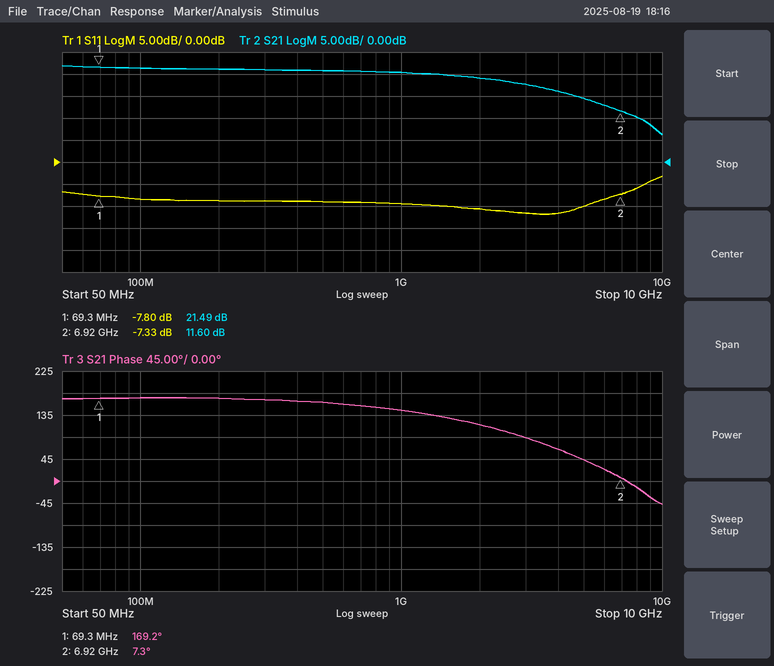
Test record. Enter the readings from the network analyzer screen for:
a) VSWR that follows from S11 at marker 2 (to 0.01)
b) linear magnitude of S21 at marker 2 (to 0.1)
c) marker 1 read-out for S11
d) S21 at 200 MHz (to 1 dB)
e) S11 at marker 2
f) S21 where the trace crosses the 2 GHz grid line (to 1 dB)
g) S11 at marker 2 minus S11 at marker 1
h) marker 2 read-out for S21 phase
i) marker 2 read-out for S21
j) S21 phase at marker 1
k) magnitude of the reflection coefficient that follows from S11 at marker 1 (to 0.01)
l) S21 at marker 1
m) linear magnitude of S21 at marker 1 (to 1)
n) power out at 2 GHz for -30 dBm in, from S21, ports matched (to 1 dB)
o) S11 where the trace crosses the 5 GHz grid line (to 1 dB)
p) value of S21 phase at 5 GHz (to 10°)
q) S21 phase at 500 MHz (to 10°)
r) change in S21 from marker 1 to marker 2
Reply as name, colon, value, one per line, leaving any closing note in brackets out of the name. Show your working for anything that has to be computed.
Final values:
VSWR that follows from S11 at marker 2: (1 + 0.4300)/(1 − 0.4300) ≈ 2.51
linear magnitude of S21 at marker 2: 10^(11.6/20) ≈ 3.8
marker 1 read-out for S11: -7.80 dB
S21 at 200 MHz: 21 dB
S11 at marker 2: -7.33 dB
S21 where the trace crosses the 2 GHz grid line: 19 dB
S11 at marker 2 minus S11 at marker 1: -7.33 − (-7.8) = 0.47 dB
marker 2 read-out for S21 phase: 7.3°
marker 2 read-out for S21: 11.60 dB
S21 phase at marker 1: 169.2°
magnitude of the reflection coefficient that follows from S11 at marker 1: 10^(-7.8/20) ≈ 0.41
S21 at marker 1: 21.49 dB
linear magnitude of S21 at marker 1: 10^(21.49/20) ≈ 12
power out at 2 GHz for -30 dBm in, from S21, ports matched: -30 dBm + (19 dB) = -11 dBm
S11 where the trace crosses the 5 GHz grid line: -10 dB
value of S21 phase at 5 GHz: 40°
S21 phase at 500 MHz: 160°
change in S21 from marker 1 to marker 2: 11.6 − (21.49) = -9.89 dB
